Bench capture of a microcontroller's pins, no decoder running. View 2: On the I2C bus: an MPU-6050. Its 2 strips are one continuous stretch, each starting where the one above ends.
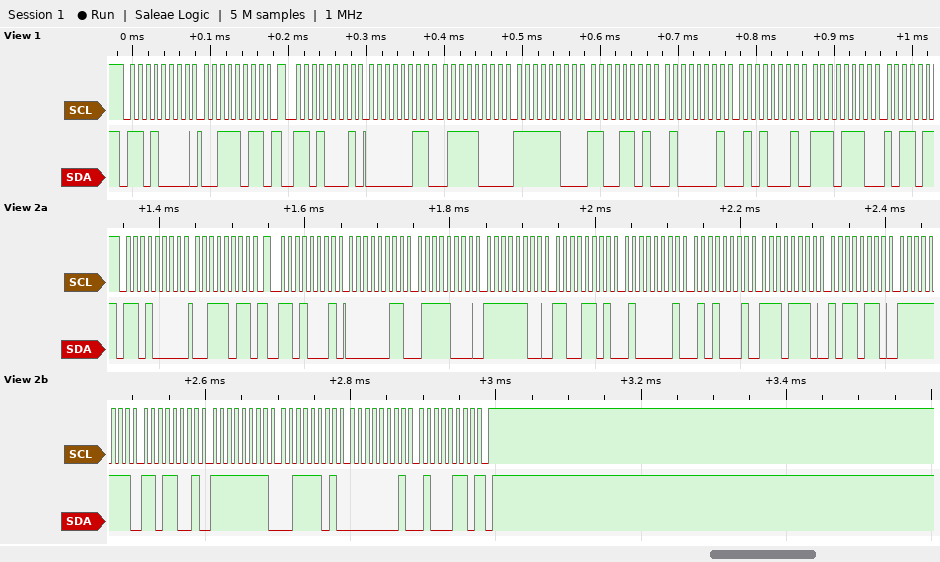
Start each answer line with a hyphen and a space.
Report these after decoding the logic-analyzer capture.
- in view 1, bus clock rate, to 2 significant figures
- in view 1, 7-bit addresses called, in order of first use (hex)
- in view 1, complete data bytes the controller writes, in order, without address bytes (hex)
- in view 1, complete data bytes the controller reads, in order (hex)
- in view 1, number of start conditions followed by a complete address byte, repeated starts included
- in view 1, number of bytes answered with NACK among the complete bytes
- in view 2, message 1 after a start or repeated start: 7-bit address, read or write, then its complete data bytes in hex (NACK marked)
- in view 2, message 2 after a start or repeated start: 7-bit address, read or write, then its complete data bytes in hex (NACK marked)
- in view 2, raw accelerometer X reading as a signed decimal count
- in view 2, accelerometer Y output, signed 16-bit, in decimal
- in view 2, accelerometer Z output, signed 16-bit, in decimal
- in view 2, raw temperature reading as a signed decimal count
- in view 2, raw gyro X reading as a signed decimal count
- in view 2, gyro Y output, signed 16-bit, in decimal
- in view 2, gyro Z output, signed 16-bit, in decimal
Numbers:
- 100 kHz
- 0x68
- 3B
- 03 78 FC CD 41 51 EE
- 2
- 0
- 0x68 write: 3B
- 0x68 read: 03 78 FC CD 41 51 EE B6 FF D9 FF 3D 01 46 NACK
- 888
- -819
- 16721
- -4426
- -39
- -195
- 326
